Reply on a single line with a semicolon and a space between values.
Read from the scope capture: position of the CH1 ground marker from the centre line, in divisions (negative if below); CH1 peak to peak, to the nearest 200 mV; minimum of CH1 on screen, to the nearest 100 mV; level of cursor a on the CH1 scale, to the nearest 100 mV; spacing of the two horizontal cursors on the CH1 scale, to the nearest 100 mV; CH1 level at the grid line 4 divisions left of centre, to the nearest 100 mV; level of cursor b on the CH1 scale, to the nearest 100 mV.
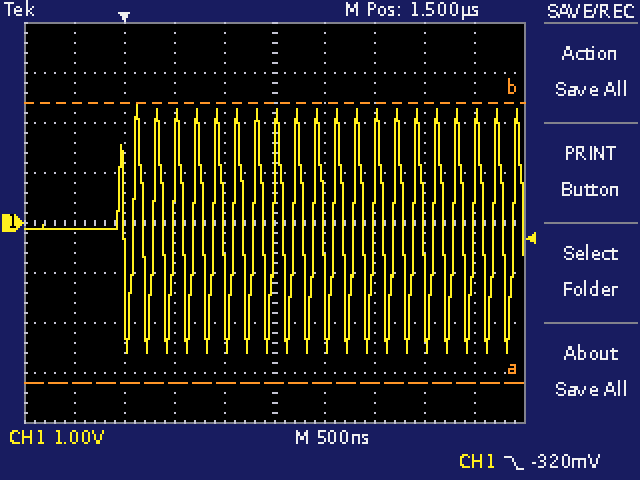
0.0 div; 5.0 V; -2.6 V; -3.2 V; 5.6 V; -100 mV; 2.4 V
